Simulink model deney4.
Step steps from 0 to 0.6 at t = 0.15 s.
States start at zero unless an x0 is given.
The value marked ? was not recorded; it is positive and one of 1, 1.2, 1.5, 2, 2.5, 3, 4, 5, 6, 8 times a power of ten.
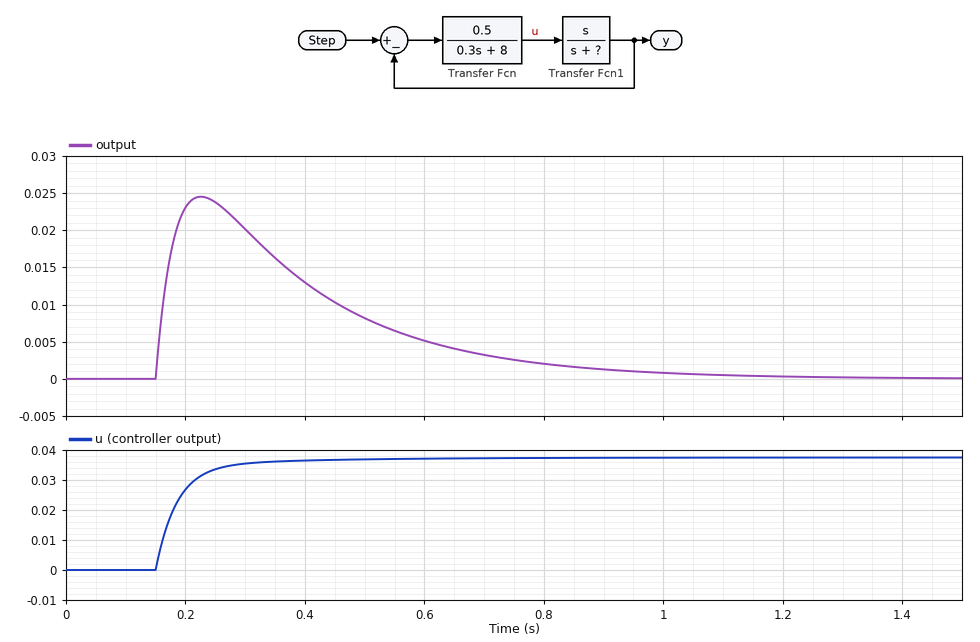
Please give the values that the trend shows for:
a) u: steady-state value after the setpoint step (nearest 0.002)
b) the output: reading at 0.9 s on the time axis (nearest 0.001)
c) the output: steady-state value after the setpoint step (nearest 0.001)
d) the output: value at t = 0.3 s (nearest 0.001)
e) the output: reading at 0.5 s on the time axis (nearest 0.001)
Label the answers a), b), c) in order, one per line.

a) 0.038
b) 0.001
c) 0.000
d) 0.020
e) 0.008
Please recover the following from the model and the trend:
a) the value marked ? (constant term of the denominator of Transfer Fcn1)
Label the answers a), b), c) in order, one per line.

a) 5
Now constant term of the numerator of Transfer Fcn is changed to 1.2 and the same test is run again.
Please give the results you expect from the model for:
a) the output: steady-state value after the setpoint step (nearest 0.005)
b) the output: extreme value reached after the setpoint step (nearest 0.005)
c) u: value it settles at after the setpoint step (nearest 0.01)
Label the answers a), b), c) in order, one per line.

a) 0.000
b) 0.055
c) 0.09
